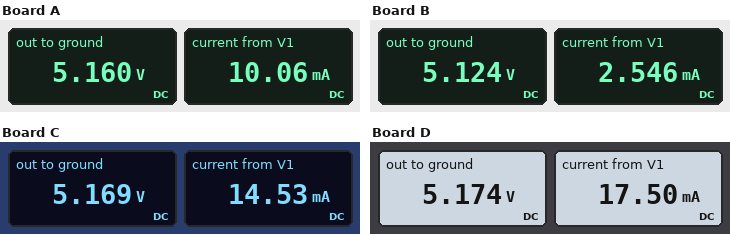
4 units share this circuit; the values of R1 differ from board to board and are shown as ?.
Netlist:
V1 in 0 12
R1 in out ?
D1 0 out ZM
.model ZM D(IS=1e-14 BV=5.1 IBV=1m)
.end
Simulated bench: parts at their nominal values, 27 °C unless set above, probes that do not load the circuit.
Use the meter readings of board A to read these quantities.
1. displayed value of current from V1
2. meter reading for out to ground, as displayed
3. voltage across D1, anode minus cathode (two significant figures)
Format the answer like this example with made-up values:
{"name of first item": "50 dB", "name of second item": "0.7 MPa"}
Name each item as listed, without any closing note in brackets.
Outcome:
{"displayed value of current from V1": "10.06 mA", "meter reading for out to ground, as displayed": "5.160 V", "voltage across D1, anode minus cathode": "-5.2 V"}
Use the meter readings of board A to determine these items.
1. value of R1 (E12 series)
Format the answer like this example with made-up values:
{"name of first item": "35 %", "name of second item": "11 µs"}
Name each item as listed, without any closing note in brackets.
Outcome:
{"value of R1": "680 Ω"}
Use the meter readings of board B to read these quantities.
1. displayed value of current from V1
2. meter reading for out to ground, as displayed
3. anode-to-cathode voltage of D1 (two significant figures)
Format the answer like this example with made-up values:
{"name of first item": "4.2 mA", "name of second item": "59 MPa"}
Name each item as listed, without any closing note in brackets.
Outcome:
{"displayed value of current from V1": "2.546 mA", "meter reading for out to ground, as displayed": "5.124 V", "anode-to-cathode voltage of D1": "-5.1 V"}
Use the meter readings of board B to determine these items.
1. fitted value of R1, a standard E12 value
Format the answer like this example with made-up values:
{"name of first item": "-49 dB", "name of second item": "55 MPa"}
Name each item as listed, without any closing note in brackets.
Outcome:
{"fitted value of R1, a standard E12 value": "2.7 kΩ"}
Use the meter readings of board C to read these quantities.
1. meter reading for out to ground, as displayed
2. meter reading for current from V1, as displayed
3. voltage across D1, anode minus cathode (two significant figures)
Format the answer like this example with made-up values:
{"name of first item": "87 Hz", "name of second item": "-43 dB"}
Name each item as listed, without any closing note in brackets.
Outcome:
{"meter reading for out to ground, as displayed": "5.169 V", "meter reading for current from V1, as displayed": "14.53 mA", "voltage across D1, anode minus cathode": "-5.2 V"}
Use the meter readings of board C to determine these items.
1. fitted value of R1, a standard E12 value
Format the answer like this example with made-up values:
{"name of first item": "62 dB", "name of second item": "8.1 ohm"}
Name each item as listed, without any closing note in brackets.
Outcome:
{"fitted value of R1, a standard E12 value": "470 Ω"}
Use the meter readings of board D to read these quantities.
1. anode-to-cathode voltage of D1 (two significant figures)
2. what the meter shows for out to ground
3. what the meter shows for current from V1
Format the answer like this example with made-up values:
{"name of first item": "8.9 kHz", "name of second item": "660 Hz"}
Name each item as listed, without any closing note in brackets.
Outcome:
{"anode-to-cathode voltage of D1": "-5.2 V", "what the meter shows for out to ground": "5.174 V", "what the meter shows for current from V1": "17.50 mA"}
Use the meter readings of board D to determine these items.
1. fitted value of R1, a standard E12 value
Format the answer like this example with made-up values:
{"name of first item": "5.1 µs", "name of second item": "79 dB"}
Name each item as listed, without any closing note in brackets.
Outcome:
{"fitted value of R1, a standard E12 value": "390 Ω"}
